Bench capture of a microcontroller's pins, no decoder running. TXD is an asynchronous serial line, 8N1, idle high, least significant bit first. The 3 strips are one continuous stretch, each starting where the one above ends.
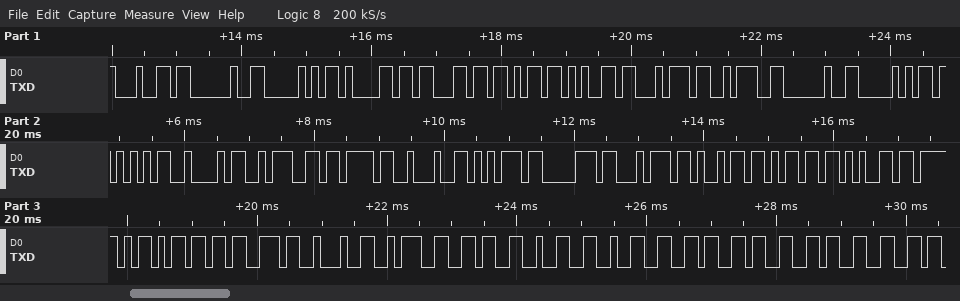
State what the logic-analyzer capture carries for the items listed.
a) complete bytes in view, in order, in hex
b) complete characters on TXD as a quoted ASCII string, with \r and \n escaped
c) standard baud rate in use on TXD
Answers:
64 20 50 61 63 6B 65 74 3A 20 50 55 42 3A 7B 22 75 70 74 69 6D 65 5F 6D 73 22 3A 36 32 32 36 33 33
"d Packet: PUB:{\"uptime_ms\":622633"
9600 baud
